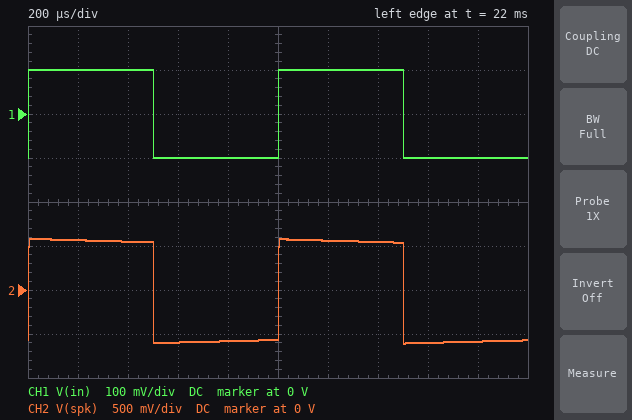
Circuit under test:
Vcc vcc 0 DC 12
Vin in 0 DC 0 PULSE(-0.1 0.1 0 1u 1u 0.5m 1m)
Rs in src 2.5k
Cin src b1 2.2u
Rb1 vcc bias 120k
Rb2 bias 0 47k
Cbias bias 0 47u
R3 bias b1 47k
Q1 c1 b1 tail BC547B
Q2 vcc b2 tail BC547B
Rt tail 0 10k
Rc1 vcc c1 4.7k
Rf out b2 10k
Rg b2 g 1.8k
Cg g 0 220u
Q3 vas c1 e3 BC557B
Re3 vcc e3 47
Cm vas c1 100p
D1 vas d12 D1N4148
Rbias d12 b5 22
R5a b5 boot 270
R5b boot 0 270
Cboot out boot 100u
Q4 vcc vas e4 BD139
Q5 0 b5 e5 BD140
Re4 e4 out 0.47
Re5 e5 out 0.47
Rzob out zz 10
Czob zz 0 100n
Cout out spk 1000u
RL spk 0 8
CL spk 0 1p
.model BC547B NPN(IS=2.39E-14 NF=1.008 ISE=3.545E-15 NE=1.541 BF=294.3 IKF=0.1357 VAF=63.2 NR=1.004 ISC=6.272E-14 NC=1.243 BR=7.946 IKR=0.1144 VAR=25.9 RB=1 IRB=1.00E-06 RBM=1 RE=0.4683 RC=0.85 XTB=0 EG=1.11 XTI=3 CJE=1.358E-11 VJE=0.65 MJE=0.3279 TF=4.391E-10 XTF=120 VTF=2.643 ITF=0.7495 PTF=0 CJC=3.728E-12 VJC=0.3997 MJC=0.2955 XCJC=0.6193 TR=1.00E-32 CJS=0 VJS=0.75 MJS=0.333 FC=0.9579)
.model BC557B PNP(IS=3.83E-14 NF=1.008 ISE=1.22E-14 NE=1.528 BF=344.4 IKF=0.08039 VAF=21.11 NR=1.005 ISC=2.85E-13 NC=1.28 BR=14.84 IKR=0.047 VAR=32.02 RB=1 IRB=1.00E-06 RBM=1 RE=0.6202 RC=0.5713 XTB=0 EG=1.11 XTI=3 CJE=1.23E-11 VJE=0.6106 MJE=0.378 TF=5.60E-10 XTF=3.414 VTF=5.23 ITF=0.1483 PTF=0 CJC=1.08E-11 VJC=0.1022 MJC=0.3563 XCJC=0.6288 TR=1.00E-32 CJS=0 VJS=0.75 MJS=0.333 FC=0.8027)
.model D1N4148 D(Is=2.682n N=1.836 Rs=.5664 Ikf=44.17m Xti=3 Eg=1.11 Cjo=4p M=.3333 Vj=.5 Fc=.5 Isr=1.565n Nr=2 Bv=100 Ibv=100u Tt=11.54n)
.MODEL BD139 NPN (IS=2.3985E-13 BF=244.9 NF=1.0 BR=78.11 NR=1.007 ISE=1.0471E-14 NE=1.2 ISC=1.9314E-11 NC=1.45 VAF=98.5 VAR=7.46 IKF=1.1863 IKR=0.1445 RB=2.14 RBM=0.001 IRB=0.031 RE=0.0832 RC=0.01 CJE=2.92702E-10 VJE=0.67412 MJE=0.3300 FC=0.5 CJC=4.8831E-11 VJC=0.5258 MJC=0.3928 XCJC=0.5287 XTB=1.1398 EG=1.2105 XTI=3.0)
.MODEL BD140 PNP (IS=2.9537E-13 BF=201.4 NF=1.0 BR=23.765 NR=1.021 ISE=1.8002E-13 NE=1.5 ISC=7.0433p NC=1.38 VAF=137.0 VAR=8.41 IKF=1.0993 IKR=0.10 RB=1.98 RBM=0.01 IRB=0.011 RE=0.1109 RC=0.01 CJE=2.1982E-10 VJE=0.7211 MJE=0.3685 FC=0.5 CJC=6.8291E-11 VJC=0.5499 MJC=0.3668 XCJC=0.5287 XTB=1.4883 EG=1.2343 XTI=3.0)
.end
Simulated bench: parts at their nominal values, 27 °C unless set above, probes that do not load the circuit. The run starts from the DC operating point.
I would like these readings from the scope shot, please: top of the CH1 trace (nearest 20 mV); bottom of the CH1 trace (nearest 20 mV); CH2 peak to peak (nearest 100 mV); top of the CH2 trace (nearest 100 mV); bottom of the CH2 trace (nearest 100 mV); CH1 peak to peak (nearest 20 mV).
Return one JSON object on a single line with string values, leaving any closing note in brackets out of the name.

{"top of the CH1 trace": "100 mV", "bottom of the CH1 trace": "-100 mV", "CH2 peak to peak": "1.2 V", "top of the CH2 trace": "600 mV", "bottom of the CH2 trace": "-600 mV", "CH1 peak to peak": "200 mV"}
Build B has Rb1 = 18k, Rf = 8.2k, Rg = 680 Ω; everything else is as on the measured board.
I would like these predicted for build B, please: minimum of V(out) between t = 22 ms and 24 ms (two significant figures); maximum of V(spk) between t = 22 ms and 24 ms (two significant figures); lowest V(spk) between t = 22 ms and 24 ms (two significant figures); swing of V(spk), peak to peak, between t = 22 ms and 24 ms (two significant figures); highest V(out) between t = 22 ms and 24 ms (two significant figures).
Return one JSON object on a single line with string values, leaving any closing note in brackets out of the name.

{"minimum of V(out) between t = 22 ms and 24 ms": "8.2 V", "maximum of V(spk) between t = 22 ms and 24 ms": "1.0 V", "lowest V(spk) between t = 22 ms and 24 ms": "-1.1 V", "swing of V(spk), peak to peak, between t = 22 ms and 24 ms": "2.1 V", "highest V(out) between t = 22 ms and 24 ms": "10 V"}
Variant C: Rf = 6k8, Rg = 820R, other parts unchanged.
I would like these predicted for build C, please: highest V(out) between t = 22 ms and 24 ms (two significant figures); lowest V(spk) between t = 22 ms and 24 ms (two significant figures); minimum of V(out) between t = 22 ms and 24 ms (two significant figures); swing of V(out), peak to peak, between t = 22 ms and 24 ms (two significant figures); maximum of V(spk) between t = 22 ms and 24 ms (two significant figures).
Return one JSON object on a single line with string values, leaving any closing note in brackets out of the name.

{"highest V(out) between t = 22 ms and 24 ms": "4.7 V", "lowest V(spk) between t = 22 ms and 24 ms": "-860 mV", "minimum of V(out) between t = 22 ms and 24 ms": "3.1 V", "swing of V(out), peak to peak, between t = 22 ms and 24 ms": "1.6 V", "maximum of V(spk) between t = 22 ms and 24 ms": "790 mV"}
